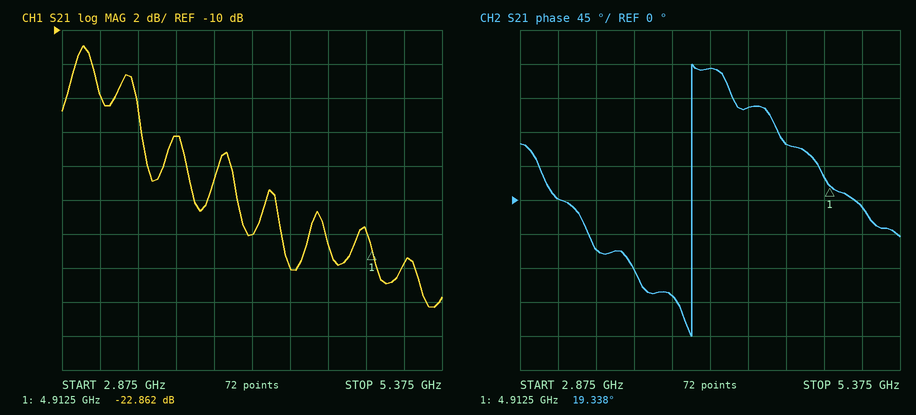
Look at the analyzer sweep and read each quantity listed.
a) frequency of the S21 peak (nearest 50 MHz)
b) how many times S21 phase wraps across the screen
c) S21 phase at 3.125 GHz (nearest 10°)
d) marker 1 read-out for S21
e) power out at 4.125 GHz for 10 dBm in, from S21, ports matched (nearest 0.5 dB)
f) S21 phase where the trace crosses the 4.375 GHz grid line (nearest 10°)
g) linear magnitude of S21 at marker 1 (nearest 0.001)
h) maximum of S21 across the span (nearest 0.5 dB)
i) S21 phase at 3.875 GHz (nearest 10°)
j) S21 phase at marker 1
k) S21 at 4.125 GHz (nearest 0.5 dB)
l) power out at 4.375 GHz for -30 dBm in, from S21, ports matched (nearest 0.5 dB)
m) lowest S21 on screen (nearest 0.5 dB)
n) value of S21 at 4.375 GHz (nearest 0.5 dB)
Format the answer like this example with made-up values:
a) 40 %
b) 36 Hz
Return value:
a) 3.00 GHz
b) 1
c) 0°
d) -22.862 dB
e) -12.0 dBm
f) 120°
g) 0.072
h) -11.0 dB
i) -130°
j) 19.338°
k) -22.0 dB
l) -54.0 dBm
m) -26.5 dB
n) -24.0 dB
